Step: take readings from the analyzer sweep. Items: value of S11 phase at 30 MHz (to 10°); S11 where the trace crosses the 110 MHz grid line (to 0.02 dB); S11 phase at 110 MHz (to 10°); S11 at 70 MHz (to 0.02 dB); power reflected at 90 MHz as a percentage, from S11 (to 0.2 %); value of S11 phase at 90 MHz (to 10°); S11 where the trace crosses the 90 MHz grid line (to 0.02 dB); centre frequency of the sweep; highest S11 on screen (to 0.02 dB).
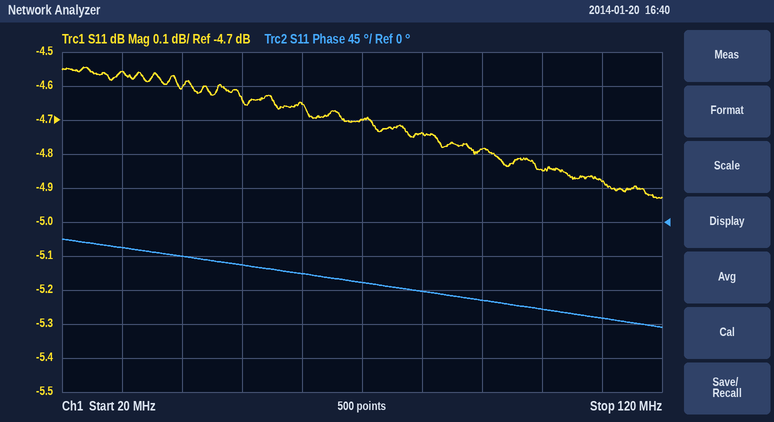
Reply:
-30°
-4.88 dB
-130°
-4.70 dB
33.2 %
-100°
-4.78 dB
70 MHz
-4.54 dB
